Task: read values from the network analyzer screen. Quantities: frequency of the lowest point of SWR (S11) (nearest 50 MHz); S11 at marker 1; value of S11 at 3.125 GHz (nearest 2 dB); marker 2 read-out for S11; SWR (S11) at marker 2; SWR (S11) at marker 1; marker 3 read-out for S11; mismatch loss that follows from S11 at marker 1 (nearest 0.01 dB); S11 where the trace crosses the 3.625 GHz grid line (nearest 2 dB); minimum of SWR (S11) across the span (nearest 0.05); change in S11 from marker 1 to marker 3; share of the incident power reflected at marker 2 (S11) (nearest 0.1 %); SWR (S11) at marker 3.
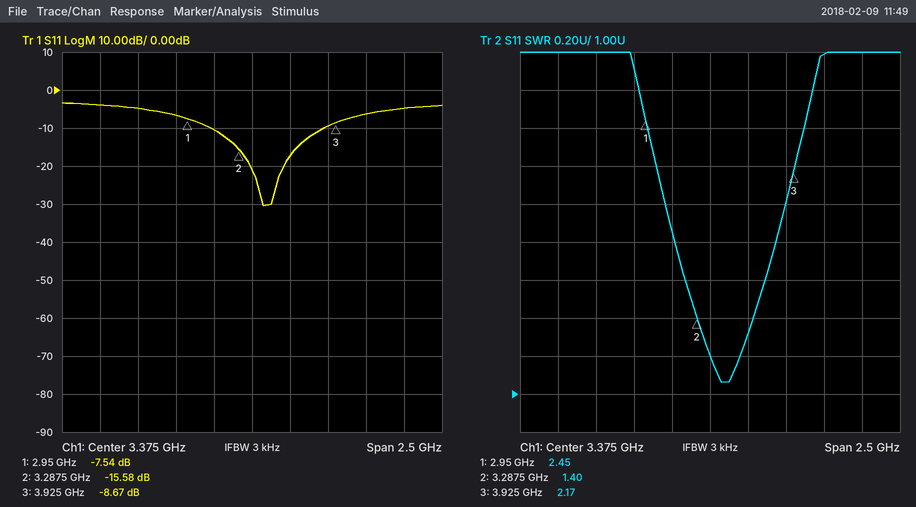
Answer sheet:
3.45 GHz
-7.54 dB
-10 dB
-15.58 dB
1.40
2.45
-8.67 dB
0.84 dB
-18 dB
1.05
-1.13 dB
2.8 %
2.17
